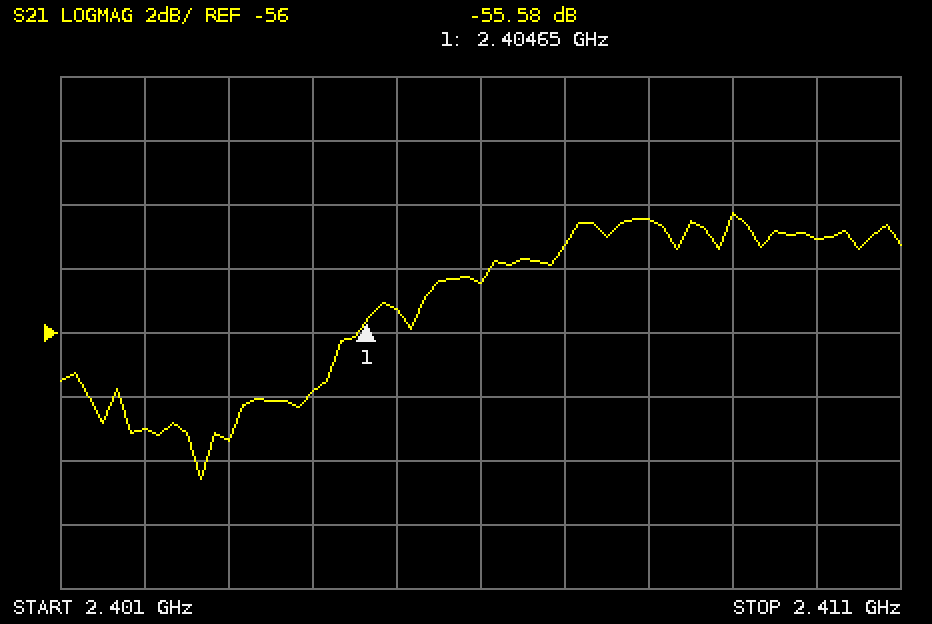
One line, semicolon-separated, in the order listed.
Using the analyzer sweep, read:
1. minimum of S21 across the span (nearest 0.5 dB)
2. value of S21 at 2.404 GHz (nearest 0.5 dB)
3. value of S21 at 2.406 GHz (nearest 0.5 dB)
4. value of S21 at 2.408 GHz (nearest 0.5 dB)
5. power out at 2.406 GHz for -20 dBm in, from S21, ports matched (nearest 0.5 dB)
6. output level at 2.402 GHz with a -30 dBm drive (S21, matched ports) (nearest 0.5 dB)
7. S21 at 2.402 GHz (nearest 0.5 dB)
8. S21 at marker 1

-60.5 dB; -58.0 dB; -54.5 dB; -52.5 dB; -74.5 dBm; -89.0 dBm; -59.0 dB; -55.58 dB
